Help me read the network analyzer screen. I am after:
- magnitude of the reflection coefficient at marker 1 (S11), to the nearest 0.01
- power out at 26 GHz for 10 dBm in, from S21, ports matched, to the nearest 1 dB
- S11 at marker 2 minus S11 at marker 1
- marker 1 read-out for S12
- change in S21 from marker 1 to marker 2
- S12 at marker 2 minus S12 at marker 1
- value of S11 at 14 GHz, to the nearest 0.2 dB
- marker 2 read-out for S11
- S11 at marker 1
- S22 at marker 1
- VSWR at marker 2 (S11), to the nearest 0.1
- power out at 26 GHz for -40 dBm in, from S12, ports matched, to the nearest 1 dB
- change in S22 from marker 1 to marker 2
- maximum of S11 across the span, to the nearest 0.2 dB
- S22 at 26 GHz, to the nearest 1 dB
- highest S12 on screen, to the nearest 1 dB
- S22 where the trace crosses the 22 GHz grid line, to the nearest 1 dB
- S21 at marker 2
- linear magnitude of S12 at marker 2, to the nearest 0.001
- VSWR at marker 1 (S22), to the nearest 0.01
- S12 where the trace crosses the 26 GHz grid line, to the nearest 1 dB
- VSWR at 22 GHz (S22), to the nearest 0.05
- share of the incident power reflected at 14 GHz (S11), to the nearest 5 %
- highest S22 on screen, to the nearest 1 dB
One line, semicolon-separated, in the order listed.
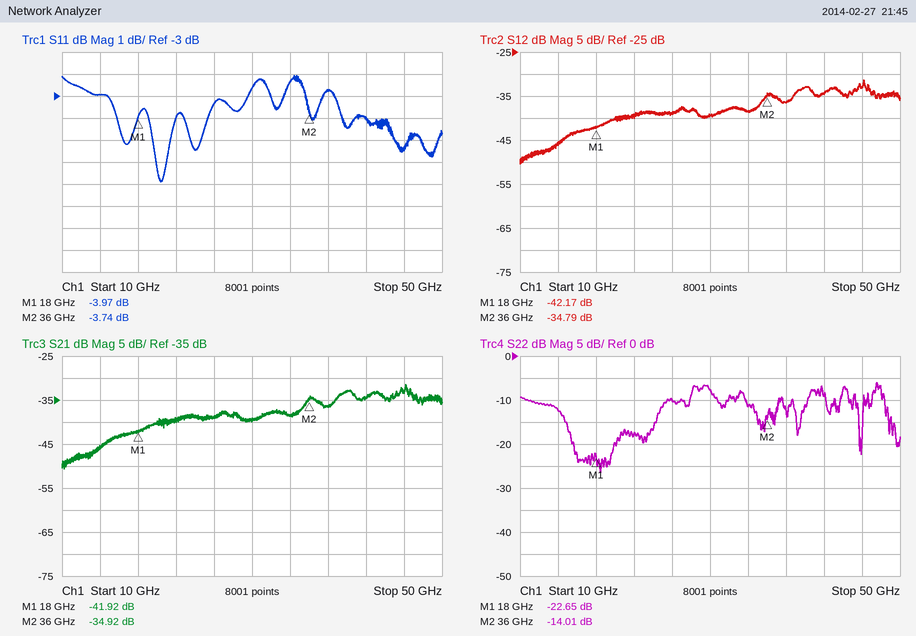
0.63; -29 dBm; 0.23 dB; -42.17 dB; 7.00 dB; 7.38 dB; -3.0 dB; -3.74 dB; -3.97 dB; -22.65 dB; 4.7; -79 dBm; 8.64 dB; -2.0 dB; -10 dB; -31 dB; -18 dB; -34.92 dB; 0.018; 1.16; -39 dB; 1.30; 50 %; -6 dB
